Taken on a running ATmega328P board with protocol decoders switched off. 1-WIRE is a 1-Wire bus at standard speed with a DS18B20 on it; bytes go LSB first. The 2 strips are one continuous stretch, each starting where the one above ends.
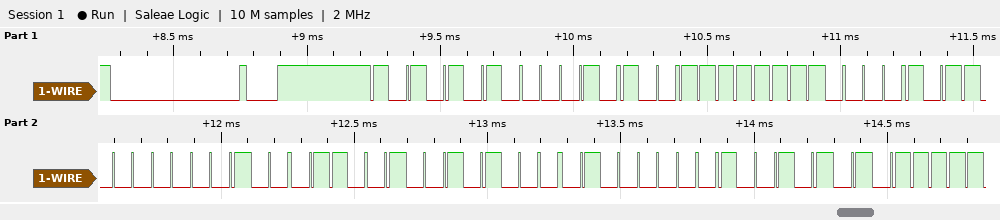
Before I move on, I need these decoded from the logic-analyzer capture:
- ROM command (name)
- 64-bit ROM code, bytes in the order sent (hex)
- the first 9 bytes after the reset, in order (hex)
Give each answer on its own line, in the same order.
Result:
Match ROM
28 FF D0 80 98 14 02 A9
55 28 FF D0 80 98 14 02 A9
